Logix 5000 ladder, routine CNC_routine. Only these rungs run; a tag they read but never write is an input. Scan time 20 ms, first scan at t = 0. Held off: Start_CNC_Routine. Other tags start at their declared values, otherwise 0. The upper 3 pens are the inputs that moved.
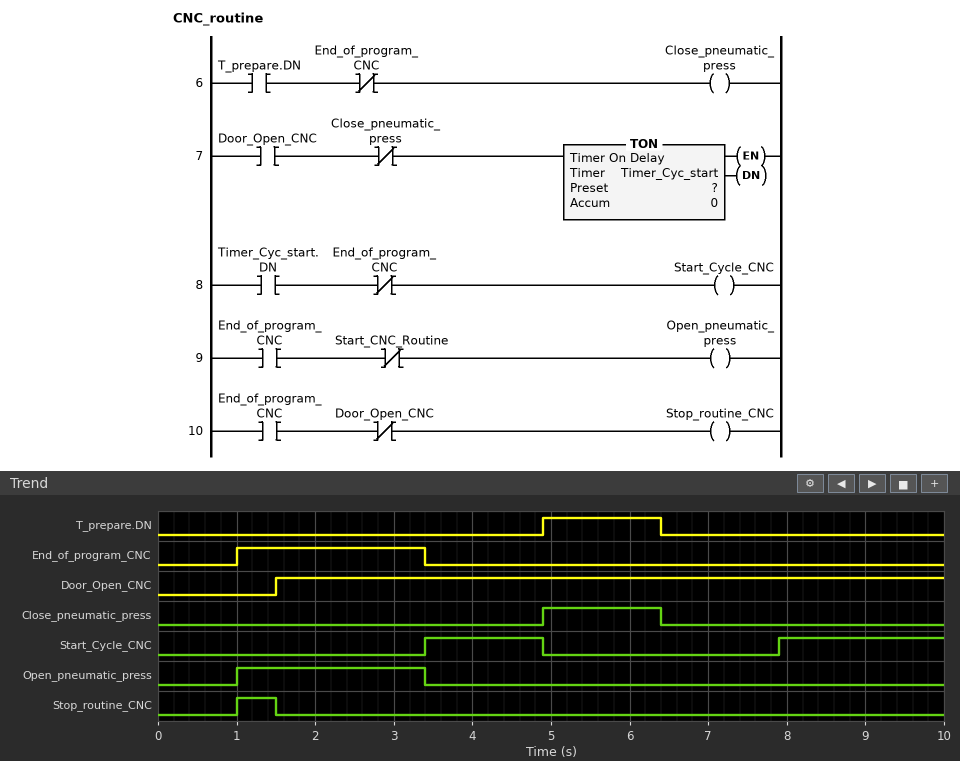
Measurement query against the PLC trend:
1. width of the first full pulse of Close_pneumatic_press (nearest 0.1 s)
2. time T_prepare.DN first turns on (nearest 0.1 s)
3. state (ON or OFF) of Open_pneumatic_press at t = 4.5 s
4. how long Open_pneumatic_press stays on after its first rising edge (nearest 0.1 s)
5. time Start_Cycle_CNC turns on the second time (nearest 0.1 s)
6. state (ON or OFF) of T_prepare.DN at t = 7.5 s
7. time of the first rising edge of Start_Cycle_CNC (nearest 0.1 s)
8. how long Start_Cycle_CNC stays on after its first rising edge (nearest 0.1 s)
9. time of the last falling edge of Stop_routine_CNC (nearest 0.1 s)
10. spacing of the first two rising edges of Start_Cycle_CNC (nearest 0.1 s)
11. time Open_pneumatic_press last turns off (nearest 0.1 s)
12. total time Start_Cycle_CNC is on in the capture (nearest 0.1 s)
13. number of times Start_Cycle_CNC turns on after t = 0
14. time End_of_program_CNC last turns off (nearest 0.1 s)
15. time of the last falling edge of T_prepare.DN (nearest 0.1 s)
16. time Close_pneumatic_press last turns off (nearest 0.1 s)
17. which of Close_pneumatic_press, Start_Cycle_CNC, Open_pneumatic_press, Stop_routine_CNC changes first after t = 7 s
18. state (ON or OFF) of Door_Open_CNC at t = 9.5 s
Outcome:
1.5 s
4.9 s
OFF
2.4 s
7.9 s
OFF
3.4 s
1.5 s
1.5 s
4.5 s
3.4 s
3.6 s
2
3.4 s
6.4 s
6.4 s
Start_Cycle_CNC
ON
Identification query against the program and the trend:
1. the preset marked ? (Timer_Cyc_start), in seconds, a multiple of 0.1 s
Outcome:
1.5 s
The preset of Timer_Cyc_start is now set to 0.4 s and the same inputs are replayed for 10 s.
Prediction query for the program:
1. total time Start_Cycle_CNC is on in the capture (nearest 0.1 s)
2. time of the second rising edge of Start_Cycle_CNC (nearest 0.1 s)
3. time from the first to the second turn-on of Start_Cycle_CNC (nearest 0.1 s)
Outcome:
4.7 s
6.8 s
3.4 s
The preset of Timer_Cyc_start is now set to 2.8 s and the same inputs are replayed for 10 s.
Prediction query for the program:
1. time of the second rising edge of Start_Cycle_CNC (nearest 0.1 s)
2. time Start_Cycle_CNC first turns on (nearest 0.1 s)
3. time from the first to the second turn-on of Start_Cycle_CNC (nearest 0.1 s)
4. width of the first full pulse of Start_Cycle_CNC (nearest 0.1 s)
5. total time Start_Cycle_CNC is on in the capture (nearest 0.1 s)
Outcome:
9.2 s
4.3 s
4.9 s
0.6 s
1.4 s
